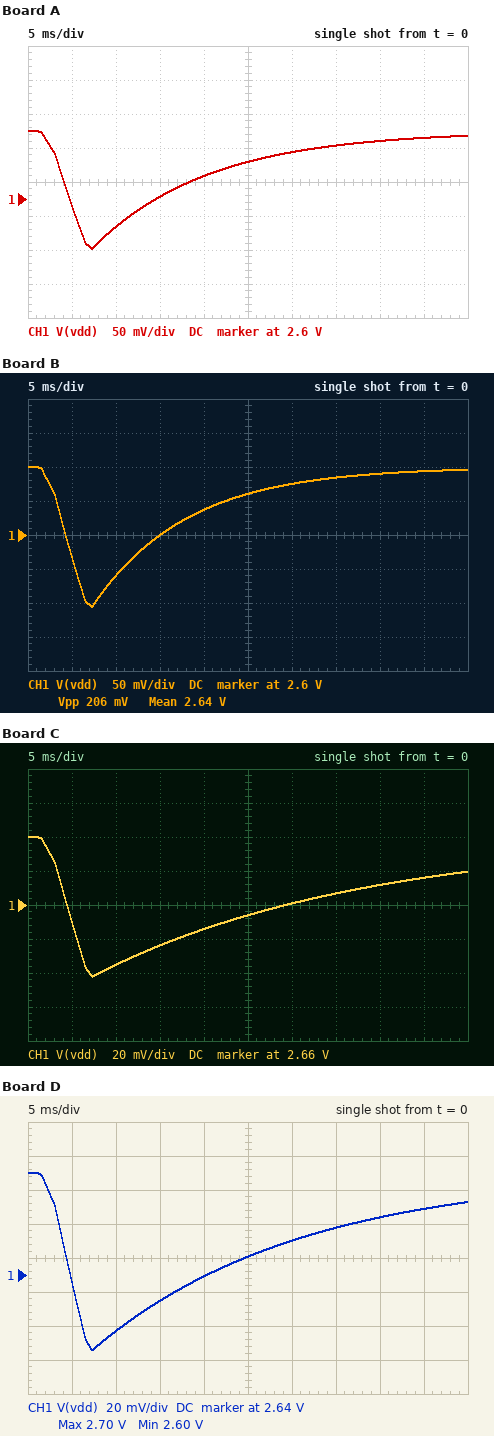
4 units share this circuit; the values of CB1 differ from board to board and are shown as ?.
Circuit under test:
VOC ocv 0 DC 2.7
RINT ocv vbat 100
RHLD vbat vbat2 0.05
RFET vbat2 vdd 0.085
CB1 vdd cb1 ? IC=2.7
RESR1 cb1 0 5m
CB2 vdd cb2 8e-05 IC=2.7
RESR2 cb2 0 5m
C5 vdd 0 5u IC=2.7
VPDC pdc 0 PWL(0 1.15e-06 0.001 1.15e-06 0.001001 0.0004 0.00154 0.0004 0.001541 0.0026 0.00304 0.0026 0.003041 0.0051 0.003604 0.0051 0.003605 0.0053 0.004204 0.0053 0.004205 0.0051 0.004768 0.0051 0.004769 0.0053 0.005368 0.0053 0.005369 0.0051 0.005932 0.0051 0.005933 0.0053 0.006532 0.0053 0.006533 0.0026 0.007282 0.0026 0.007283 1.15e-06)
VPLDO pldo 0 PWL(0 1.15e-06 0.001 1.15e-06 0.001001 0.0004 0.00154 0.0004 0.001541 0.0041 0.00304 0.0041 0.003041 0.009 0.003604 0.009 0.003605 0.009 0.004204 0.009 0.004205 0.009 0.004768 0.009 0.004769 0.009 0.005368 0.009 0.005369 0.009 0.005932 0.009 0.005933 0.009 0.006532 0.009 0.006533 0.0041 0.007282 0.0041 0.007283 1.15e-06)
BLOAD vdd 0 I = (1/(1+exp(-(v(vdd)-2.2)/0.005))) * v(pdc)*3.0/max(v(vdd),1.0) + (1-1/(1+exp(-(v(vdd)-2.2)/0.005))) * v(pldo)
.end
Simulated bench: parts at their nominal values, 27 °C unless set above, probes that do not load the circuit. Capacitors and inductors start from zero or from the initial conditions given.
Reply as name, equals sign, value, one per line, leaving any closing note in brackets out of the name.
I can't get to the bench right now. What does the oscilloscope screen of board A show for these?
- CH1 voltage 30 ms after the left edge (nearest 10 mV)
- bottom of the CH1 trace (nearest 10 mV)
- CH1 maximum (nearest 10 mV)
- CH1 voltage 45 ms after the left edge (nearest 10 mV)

CH1 voltage 30 ms after the left edge = 2.67 V
bottom of the CH1 trace = 2.53 V
CH1 maximum = 2.70 V
CH1 voltage 45 ms after the left edge = 2.69 V
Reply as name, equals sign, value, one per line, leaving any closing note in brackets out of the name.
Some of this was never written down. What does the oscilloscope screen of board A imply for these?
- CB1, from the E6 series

CB1, from the E6 series = 47 µF
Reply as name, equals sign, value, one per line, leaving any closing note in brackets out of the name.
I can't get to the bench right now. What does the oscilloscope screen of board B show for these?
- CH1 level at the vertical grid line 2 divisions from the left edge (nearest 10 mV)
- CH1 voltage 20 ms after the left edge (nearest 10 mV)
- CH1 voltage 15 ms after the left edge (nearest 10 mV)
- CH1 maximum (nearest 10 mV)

CH1 level at the vertical grid line 2 divisions from the left edge = 2.54 V
CH1 voltage 20 ms after the left edge = 2.64 V
CH1 voltage 15 ms after the left edge = 2.60 V
CH1 maximum = 2.70 V
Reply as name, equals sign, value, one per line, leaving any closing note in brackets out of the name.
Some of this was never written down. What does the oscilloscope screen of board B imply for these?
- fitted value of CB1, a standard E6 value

fitted value of CB1, a standard E6 value = 22 µF
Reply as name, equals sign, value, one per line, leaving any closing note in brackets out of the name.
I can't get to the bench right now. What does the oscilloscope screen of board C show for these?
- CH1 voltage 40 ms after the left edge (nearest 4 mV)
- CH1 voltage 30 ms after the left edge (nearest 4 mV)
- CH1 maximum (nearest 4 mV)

CH1 voltage 40 ms after the left edge = 2.672 V
CH1 voltage 30 ms after the left edge = 2.660 V
CH1 maximum = 2.700 V
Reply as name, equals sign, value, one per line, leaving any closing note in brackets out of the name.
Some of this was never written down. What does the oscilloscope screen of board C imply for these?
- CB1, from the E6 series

CB1, from the E6 series = 220 µF
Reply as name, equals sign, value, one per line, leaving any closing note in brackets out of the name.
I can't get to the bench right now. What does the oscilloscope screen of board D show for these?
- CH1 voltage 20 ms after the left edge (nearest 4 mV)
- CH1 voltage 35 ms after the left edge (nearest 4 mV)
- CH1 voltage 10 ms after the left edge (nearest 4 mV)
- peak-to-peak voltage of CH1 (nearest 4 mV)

CH1 voltage 20 ms after the left edge = 2.640 V
CH1 voltage 35 ms after the left edge = 2.668 V
CH1 voltage 10 ms after the left edge = 2.608 V
peak-to-peak voltage of CH1 = 104 mV
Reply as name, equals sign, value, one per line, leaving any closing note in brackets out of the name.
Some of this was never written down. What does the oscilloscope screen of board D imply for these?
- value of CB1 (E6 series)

value of CB1 = 150 µF
